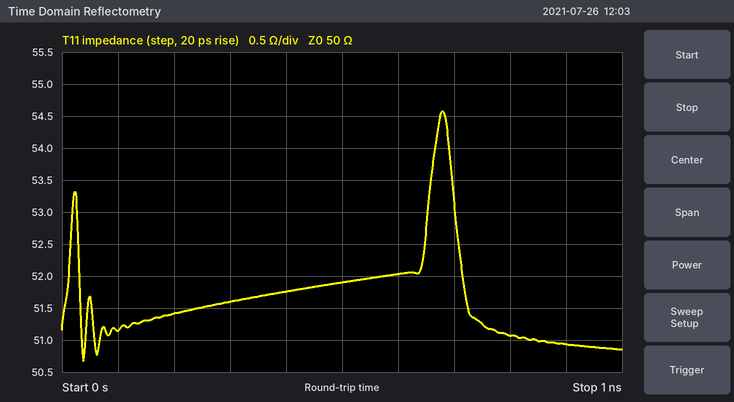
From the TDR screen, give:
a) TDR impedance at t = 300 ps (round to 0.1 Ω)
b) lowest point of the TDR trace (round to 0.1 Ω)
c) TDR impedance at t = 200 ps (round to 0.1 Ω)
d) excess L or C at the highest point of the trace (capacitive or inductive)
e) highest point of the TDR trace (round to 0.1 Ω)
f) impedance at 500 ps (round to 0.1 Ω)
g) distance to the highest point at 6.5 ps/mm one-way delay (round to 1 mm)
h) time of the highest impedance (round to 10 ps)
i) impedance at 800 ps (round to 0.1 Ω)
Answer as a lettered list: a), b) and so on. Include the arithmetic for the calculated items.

a) 51.6 Ω
b) 50.7 Ω
c) 51.4 Ω
d) inductive
e) 54.6 Ω
f) 51.9 Ω
g) 680 ps / 2 / 6.5 ps/mm ≈ 52 mm
h) 680 ps
i) 51.1 Ω
